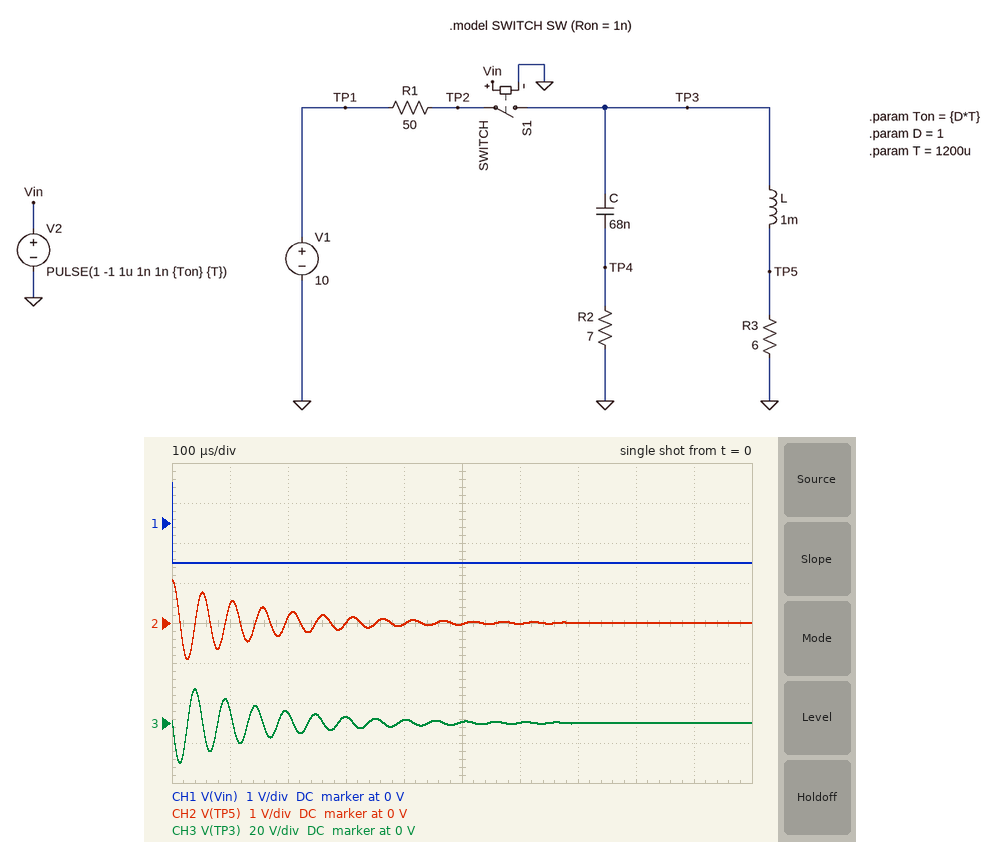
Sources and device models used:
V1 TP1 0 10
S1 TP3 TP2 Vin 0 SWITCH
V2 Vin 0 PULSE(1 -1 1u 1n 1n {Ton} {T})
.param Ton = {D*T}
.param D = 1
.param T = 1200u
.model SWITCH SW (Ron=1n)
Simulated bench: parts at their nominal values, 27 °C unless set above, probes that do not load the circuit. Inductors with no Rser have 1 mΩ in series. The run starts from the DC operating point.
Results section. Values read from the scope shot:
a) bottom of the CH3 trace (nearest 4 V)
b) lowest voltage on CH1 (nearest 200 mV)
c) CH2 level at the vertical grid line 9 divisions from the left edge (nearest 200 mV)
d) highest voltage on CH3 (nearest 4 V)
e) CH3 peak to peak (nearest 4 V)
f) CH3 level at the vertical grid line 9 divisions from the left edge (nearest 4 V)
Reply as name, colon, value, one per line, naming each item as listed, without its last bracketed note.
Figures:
bottom of the CH3 trace: -20 V
lowest voltage on CH1: -1.0 V
CH2 level at the vertical grid line 9 divisions from the left edge: 0 V
highest voltage on CH3: 16 V
CH3 peak to peak: 36 V
CH3 level at the vertical grid line 9 divisions from the left edge: 0 V
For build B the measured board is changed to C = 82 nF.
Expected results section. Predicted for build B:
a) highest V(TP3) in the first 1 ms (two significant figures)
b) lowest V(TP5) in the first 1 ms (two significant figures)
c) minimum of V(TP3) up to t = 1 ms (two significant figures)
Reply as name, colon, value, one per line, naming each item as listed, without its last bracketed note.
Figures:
highest V(TP3) in the first 1 ms: 15 V
lowest V(TP5) in the first 1 ms: -890 mV
minimum of V(TP3) up to t = 1 ms: -18 V
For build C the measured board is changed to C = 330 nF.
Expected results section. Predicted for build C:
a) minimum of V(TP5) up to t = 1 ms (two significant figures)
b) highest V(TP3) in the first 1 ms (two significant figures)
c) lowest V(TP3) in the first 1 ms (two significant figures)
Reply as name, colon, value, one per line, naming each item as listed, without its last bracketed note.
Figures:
minimum of V(TP5) up to t = 1 ms: -740 mV
highest V(TP3) in the first 1 ms: 5.6 V
lowest V(TP3) in the first 1 ms: -8.2 V
